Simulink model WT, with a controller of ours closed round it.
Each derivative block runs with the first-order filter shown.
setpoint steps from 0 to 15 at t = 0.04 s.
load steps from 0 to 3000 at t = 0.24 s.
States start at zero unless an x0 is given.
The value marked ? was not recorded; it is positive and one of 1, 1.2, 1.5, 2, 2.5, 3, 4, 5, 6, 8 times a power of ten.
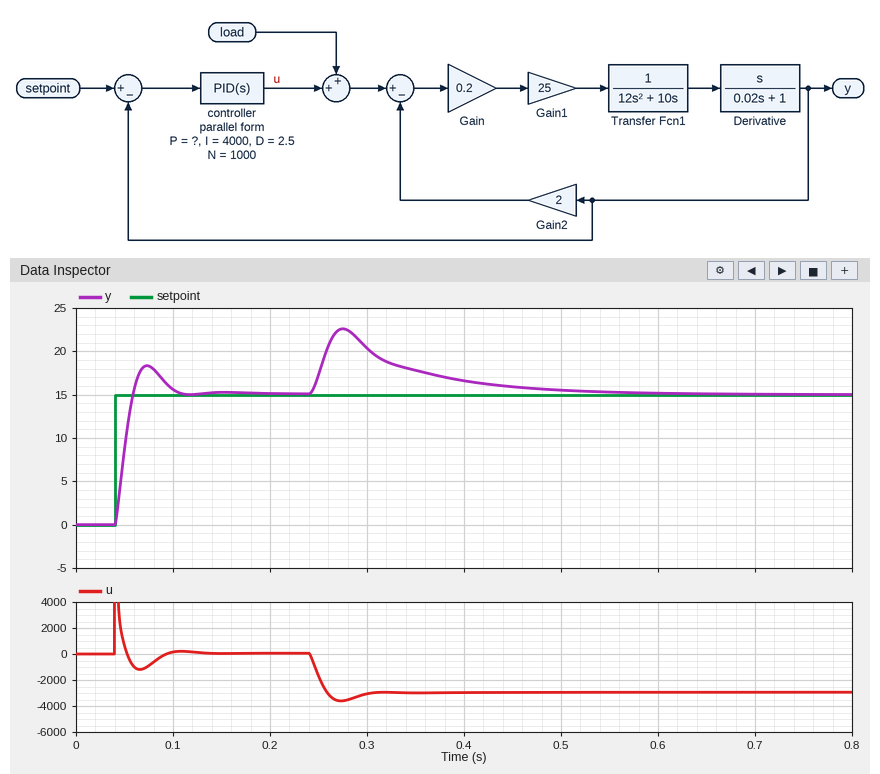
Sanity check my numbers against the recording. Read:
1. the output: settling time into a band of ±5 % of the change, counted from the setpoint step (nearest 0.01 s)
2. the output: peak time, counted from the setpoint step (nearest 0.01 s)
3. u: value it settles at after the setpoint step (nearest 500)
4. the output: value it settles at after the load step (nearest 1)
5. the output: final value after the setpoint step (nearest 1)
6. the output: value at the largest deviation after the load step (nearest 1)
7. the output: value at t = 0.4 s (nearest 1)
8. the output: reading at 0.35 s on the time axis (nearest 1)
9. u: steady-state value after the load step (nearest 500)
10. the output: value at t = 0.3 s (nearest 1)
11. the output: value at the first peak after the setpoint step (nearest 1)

0.06 s
0.03 s
0
15
15
23
17
18
-3000
20
18
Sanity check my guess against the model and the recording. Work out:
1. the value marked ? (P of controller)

400
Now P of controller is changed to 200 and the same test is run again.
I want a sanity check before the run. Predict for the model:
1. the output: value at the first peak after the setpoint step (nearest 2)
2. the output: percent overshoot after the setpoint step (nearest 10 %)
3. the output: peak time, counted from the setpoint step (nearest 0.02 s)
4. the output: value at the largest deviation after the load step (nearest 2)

18
20 %
0.06 s
26
